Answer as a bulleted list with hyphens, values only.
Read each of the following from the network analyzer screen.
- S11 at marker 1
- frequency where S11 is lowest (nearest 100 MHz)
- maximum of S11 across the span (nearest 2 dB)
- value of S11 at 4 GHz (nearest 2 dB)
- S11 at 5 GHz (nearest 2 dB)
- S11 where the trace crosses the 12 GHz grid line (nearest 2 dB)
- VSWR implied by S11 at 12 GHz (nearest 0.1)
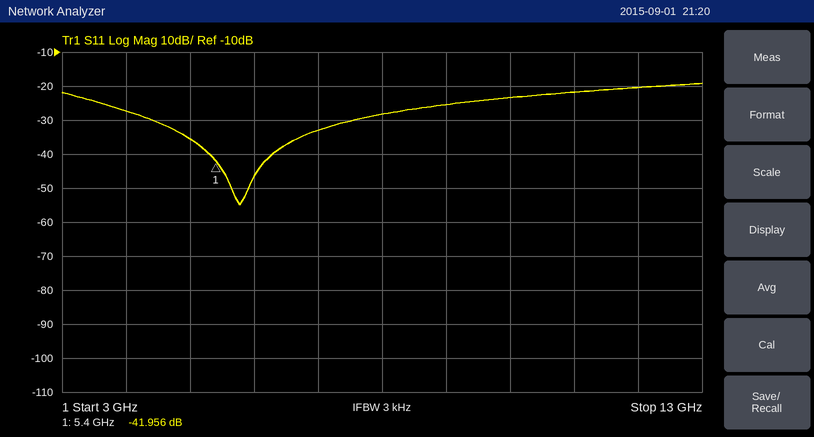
- -41.956 dB
- 5.8 GHz
- -20 dB
- -28 dB
- -36 dB
- -20 dB
- 1.2
